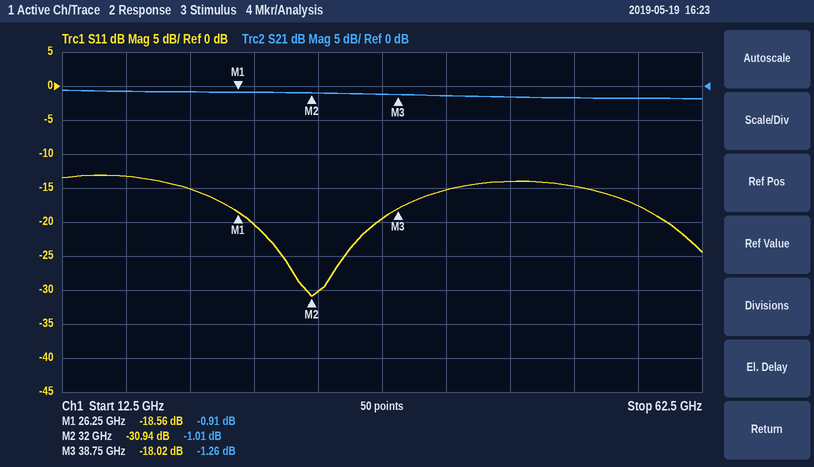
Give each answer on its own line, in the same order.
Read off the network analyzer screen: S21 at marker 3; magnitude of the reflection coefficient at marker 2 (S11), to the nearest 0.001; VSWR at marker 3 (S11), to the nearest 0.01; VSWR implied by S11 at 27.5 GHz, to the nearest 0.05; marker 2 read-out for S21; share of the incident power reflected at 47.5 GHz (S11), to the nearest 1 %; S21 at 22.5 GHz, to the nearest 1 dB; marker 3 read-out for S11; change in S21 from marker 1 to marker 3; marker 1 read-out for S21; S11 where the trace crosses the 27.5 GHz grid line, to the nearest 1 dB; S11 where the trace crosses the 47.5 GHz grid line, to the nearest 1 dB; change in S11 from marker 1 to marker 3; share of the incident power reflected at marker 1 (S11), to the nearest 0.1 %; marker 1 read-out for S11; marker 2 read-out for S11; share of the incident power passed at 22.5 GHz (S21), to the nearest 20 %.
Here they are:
-1.26 dB
0.028
1.29
1.20
-1.01 dB
4 %
-1 dB
-18.02 dB
-0.35 dB
-0.91 dB
-20 dB
-14 dB
0.54 dB
1.4 %
-18.56 dB
-30.94 dB
80 %
